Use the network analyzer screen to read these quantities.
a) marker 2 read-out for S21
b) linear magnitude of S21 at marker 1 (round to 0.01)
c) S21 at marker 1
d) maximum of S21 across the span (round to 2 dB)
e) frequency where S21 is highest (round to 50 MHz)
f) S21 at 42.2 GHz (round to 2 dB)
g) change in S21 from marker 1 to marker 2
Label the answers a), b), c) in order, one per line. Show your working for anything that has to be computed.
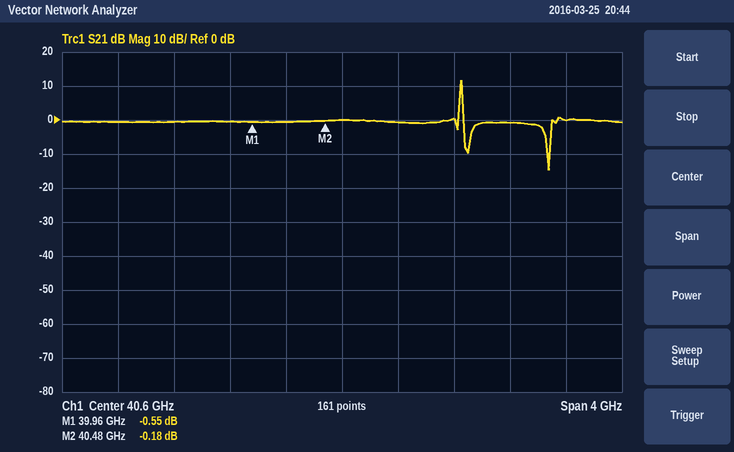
a) -0.18 dB
b) 10^(-0.55/20) ≈ 0.94
c) -0.55 dB
d) 12 dB
e) 41.45 GHz
f) 0 dB
g) -0.18 − (-0.55) = 0.37 dB
